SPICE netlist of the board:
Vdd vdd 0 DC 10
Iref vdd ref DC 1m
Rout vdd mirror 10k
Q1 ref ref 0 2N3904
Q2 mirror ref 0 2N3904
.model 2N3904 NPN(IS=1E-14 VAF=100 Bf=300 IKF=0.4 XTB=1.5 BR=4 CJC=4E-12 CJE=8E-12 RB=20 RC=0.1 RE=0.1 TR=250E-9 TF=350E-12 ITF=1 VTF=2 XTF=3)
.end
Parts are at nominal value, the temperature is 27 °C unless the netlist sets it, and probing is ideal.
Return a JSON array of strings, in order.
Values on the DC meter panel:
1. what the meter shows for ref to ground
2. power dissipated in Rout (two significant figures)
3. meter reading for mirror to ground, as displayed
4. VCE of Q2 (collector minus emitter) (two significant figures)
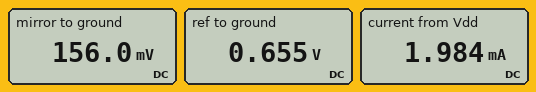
["0.655 V", "9.7 mW", "156.0 mV", "160 mV"]
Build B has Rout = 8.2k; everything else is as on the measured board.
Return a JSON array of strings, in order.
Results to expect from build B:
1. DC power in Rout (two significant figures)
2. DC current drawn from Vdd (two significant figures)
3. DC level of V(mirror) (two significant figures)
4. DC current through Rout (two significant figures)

["8.3 mW", "2.0 mA", "1.8 V", "1.0 mA"]
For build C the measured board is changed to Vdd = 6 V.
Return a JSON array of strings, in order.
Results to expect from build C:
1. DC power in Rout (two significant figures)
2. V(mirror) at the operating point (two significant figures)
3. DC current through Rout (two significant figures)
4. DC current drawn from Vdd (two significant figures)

["3.6 mW", "35 mV", "600 µA", "1.6 mA"]
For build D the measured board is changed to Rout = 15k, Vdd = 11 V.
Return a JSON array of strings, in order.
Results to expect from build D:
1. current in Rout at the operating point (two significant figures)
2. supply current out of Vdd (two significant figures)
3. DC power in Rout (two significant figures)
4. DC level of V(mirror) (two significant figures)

["730 µA", "1.7 mA", "8.0 mW", "47 mV"]
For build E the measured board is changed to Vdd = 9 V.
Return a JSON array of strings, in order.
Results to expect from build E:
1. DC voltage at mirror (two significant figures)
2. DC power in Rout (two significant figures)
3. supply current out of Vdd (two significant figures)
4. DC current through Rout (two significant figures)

["74 mV", "8.0 mW", "1.9 mA", "890 µA"]
